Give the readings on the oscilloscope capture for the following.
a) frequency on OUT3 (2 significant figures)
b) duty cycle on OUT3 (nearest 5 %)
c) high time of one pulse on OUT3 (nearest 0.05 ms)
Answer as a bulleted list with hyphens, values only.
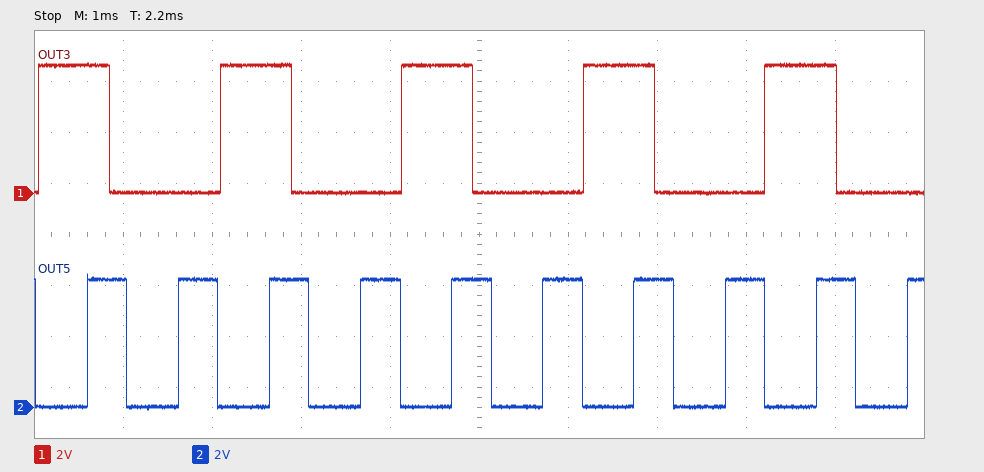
- 490 Hz
- 40 %
- 0.80 ms
